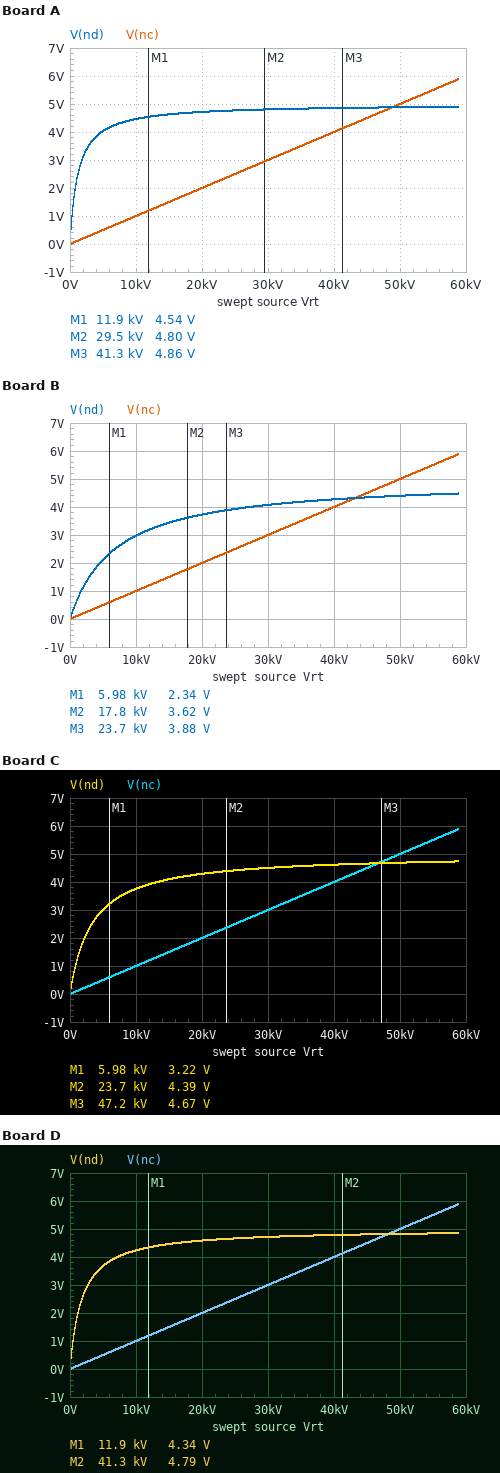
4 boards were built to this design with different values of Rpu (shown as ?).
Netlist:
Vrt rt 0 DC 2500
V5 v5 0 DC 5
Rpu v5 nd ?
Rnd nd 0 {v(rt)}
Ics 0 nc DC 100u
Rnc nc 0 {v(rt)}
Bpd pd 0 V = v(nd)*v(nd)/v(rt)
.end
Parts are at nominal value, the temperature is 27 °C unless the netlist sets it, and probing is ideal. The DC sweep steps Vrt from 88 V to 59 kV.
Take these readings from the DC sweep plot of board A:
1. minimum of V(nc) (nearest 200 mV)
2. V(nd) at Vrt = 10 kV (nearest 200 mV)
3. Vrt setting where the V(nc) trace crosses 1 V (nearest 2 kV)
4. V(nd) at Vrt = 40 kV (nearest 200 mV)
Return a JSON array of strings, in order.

["0 V", "4.4 V", "10 kV", "4.8 V"]
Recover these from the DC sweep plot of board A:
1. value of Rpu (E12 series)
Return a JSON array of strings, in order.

["1.2 kΩ"]
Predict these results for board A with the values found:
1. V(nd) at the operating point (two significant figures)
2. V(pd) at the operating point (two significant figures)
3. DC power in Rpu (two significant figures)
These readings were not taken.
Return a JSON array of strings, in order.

["3.4 V", "4.6 mV", "2.2 mW"]
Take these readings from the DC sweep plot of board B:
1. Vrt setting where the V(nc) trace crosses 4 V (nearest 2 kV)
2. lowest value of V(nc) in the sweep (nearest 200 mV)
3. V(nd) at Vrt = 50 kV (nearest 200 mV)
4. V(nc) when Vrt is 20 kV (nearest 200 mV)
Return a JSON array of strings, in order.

["40 kV", "0 V", "4.4 V", "2.0 V"]
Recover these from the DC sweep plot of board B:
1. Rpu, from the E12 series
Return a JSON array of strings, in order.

["6.8 kΩ"]
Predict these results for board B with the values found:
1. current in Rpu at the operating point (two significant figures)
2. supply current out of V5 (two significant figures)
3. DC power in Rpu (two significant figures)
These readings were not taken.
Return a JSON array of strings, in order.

["540 µA", "540 µA", "2.0 mW"]
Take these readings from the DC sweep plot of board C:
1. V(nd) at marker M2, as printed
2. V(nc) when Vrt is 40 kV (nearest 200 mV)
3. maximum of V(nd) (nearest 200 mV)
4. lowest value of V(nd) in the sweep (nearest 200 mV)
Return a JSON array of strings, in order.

["4.39 V", "4.0 V", "4.8 V", "200 mV"]
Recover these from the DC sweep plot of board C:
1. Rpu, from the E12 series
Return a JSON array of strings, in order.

["3.3 kΩ"]
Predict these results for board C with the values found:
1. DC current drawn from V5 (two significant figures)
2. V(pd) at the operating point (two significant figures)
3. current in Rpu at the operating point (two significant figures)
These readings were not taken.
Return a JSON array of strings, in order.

["860 µA", "1.9 mV", "860 µA"]
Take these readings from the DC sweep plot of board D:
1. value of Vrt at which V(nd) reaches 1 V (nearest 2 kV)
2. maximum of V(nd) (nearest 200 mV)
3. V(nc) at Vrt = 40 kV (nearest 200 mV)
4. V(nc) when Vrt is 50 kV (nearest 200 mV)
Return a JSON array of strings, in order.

["0 V", "4.8 V", "4.0 V", "5.0 V"]
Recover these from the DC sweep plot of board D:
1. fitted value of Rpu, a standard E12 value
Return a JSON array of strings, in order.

["1.8 kΩ"]
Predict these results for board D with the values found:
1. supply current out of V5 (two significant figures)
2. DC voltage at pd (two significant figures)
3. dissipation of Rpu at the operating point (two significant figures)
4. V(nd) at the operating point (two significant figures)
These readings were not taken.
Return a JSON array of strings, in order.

["1.2 mA", "3.4 mV", "2.4 mW", "2.9 V"]
